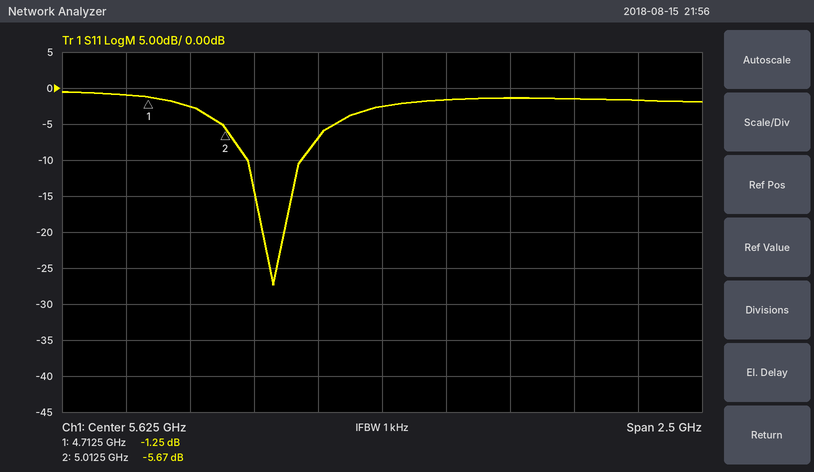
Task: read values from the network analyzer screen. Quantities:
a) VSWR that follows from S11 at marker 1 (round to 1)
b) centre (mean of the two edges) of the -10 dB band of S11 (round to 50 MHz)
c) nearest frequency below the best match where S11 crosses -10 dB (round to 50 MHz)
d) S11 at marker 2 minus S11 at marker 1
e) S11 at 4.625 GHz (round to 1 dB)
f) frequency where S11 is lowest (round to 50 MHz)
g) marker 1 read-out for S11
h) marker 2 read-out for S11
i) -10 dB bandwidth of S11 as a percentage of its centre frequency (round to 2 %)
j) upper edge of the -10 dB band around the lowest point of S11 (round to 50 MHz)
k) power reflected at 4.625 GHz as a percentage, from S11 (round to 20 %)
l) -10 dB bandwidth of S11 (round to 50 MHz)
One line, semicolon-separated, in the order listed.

14; 5.20 GHz; 5.10 GHz; -4.42 dB; -1 dB; 5.20 GHz; -1.25 dB; -5.67 dB; 4 %; 5.30 GHz; 80 %; 200 MHz
